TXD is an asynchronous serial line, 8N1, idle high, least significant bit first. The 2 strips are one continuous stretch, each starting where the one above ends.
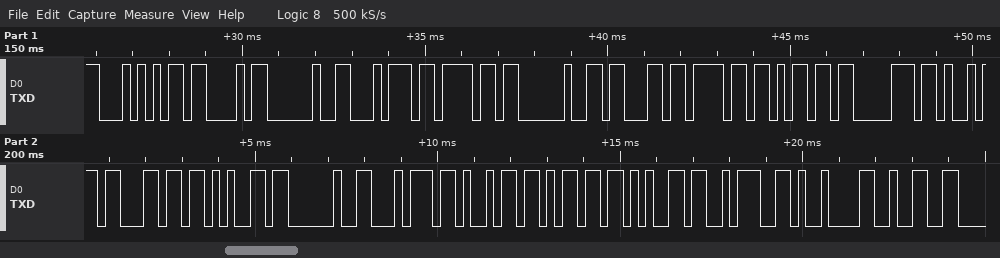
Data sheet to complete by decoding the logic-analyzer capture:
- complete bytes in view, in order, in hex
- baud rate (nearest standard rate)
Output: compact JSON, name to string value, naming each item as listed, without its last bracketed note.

{"complete bytes in view, in order, in hex": "54 43 20 74 6F 20 63 6F 6D 70 69 6C 65 20 74 69 6D 65 3A 09 32", "baud rate": "4800 baud"}
